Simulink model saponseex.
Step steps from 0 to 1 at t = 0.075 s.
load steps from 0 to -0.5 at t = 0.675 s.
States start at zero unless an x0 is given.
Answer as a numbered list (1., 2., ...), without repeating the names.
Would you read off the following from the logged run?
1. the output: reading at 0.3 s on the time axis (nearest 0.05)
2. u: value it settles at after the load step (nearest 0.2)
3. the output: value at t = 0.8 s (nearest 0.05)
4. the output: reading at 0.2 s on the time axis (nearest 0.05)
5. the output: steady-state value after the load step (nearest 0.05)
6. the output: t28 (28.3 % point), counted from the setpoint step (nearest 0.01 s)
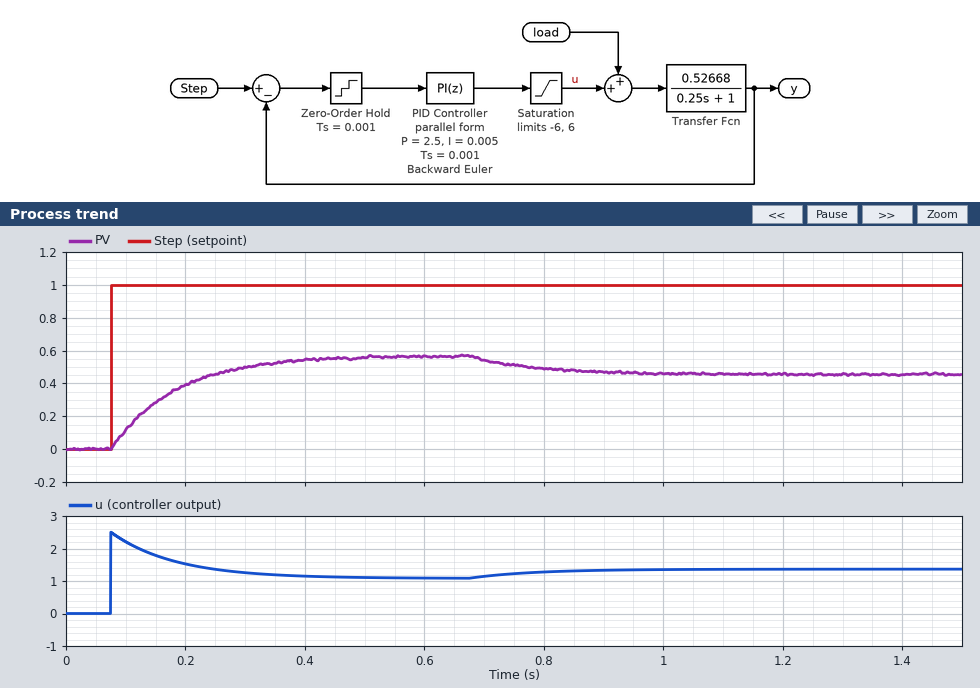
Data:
1. 0.50
2. 1.4
3. 0.50
4. 0.40
5. 0.45
6. 0.04 s
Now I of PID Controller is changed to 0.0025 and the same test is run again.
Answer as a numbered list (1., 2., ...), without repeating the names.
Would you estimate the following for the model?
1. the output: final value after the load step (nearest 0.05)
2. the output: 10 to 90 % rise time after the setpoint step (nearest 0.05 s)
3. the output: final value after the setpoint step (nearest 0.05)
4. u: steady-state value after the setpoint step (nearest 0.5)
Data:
1. 0.45
2. 0.25 s
3. 0.55
4. 1.0
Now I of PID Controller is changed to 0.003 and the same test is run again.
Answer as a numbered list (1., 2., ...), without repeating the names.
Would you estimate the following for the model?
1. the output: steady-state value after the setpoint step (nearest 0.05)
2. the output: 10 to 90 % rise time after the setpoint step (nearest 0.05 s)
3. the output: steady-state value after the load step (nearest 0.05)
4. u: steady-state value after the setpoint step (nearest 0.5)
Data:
1. 0.55
2. 0.25 s
3. 0.45
4. 1.0
